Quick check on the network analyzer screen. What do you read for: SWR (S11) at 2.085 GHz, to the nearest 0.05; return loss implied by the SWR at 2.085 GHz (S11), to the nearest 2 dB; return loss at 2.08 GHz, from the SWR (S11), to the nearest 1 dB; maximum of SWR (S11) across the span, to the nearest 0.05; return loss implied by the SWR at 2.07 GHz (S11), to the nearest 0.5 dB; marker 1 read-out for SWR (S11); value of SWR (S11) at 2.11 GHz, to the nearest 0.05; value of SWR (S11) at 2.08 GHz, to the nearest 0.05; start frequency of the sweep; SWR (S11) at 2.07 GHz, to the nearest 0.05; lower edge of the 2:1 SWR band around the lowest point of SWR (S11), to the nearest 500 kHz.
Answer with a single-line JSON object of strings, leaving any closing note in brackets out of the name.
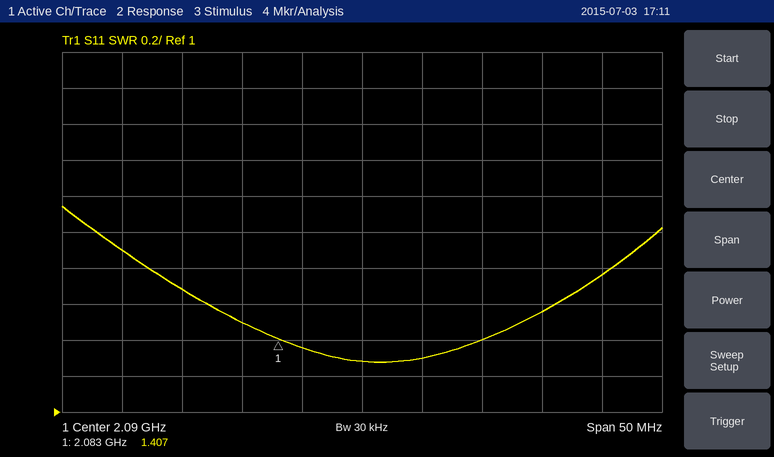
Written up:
{"SWR (S11) at 2.085 GHz, to the nearest 0.05": "1.35", "return loss implied by the SWR at 2.085 GHz (S11), to the nearest 2 dB": "16 dB", "return loss at 2.08 GHz, from the SWR (S11), to the nearest 1 dB": "14 dB", "maximum of SWR (S11) across the span, to the nearest 0.05": "2.15", "return loss implied by the SWR at 2.07 GHz (S11), to the nearest 0.5 dB": "10.0 dB", "marker 1 read-out for SWR": "1.407", "value of SWR (S11) at 2.11 GHz, to the nearest 0.05": "1.75", "value of SWR (S11) at 2.08 GHz, to the nearest 0.05": "1.50", "start frequency of the sweep": "2.065 GHz", "SWR (S11) at 2.07 GHz, to the nearest 0.05": "1.90", "lower edge of the 2:1 SWR band around the lowest point of SWR (S11), to the nearest 500 kHz": "2.0680 GHz"}
